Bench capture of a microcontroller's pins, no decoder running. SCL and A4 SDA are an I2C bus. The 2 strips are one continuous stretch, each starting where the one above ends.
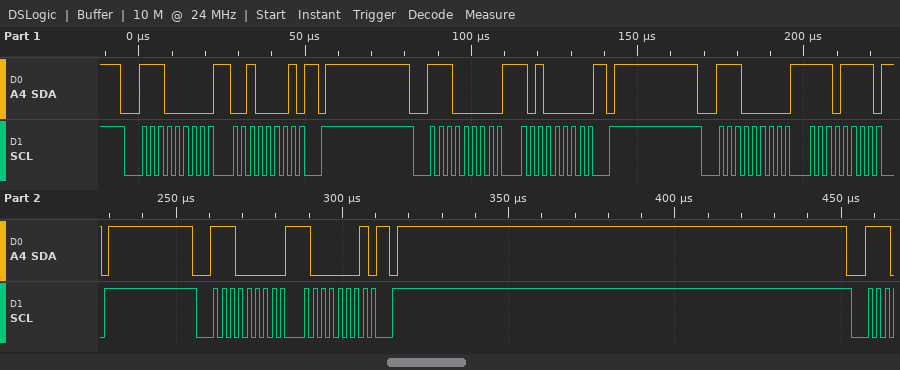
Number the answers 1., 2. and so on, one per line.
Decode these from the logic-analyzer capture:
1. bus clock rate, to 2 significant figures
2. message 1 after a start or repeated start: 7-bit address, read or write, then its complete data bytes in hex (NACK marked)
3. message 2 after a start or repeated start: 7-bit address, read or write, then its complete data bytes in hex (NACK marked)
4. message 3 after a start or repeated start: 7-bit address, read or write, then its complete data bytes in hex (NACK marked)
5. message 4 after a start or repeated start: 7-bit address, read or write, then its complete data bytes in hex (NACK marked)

1. 400 kHz
2. 0x70 write: 21
3. 0x70 write: A0
4. 0x70 write: EF
5. 0x70 write: 81
